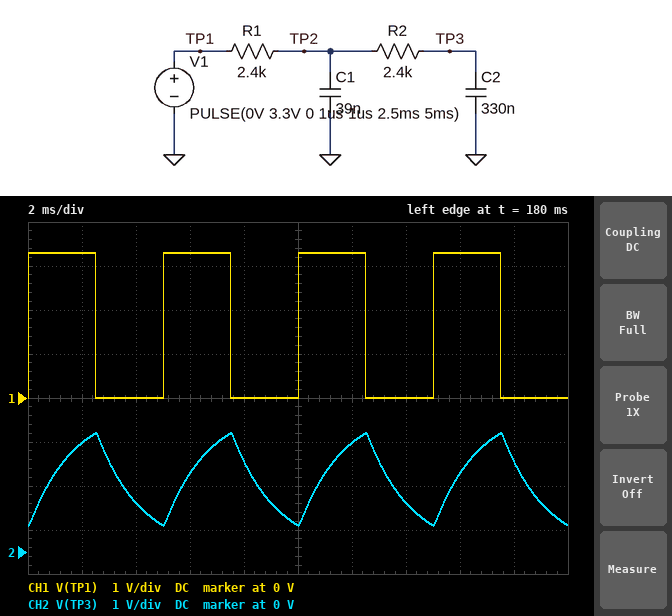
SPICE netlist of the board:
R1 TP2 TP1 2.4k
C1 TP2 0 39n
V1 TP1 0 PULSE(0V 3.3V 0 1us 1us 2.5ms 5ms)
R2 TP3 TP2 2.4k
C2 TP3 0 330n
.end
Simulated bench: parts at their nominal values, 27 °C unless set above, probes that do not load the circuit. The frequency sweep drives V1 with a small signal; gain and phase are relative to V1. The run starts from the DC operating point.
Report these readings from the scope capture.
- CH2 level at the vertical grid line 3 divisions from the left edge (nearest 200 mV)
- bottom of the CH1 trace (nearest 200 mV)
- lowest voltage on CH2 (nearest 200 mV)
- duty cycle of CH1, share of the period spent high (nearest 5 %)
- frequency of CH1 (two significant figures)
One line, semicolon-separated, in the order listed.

1.8 V; 0 V; 600 mV; 50 %; 200 Hz
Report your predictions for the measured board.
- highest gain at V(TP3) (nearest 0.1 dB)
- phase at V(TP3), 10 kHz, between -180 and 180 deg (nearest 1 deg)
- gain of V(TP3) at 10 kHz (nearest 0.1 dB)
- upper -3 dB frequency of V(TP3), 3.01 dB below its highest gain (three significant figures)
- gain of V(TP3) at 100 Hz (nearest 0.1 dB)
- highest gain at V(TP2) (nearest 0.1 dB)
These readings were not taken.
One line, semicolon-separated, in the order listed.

0 dB; -160 deg; -49.8 dB; 97.4 Hz; -3.1 dB; 0 dB
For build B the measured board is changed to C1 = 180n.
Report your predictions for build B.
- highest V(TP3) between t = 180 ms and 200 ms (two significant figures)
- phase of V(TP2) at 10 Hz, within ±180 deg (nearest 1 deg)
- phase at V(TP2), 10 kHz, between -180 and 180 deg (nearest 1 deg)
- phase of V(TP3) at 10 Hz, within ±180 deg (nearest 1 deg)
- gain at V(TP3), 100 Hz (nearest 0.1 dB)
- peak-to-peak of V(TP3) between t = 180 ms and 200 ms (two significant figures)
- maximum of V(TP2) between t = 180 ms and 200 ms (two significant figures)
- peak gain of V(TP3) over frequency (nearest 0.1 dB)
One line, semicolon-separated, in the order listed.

2.6 V; -4 deg; -86 deg; -7 deg; -3.7 dB; 1.8 V; 2.9 V; 0 dB
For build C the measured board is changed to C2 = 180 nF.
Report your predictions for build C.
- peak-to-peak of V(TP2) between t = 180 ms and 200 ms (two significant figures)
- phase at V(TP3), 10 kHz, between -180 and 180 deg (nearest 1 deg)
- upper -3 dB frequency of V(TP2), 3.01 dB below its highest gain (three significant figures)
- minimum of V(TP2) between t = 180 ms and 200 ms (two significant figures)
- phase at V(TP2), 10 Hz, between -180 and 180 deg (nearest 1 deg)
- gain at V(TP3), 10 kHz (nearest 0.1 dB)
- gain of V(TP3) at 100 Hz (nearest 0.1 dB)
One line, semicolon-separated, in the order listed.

3.1 V; -159 deg; 233 Hz; 110 mV; -2 deg; -44.6 dB; -1.2 dB
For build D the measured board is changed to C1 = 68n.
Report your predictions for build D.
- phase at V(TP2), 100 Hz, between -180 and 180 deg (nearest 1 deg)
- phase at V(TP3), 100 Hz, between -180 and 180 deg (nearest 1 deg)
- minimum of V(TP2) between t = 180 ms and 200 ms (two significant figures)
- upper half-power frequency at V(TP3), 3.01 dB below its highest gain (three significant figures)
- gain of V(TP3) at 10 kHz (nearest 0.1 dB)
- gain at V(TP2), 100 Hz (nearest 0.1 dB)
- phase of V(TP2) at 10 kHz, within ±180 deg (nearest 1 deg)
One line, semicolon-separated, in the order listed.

-23 deg; -49 deg; 330 mV; 95.1 Hz; -54.3 dB; -2.3 dB; -79 deg
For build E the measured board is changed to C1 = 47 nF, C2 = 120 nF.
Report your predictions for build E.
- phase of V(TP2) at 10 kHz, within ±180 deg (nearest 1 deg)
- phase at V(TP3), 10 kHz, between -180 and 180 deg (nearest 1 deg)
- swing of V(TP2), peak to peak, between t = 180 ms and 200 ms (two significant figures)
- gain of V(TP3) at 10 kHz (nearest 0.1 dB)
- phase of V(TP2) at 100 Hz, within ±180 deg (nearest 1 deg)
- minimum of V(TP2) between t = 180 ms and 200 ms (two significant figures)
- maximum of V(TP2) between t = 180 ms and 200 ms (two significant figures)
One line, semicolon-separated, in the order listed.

-74 deg; -161 deg; 3.2 V; -42.6 dB; -13 deg; 38 mV; 3.3 V
